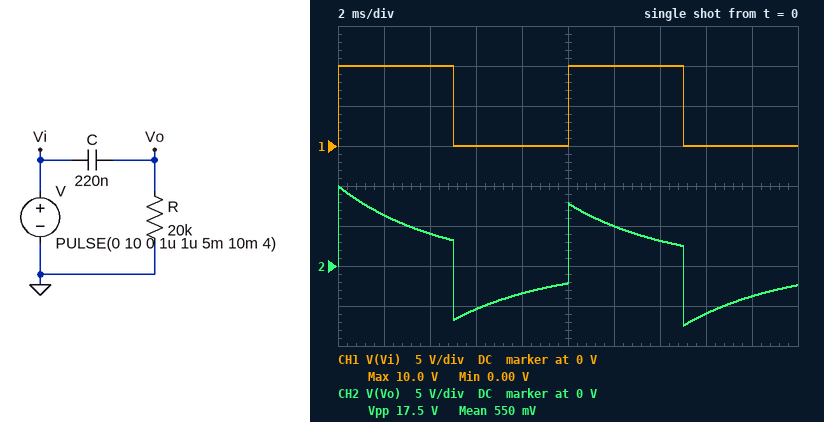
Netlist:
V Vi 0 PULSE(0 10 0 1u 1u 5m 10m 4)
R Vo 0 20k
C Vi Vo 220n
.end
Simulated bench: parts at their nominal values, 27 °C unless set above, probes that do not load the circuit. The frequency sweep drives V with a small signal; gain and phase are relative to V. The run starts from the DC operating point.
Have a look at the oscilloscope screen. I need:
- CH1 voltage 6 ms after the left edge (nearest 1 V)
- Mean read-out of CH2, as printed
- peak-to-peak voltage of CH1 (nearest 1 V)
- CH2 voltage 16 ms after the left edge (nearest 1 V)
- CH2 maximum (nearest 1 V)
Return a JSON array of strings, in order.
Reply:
["0 V", "550 mV", "10 V", "-6 V", "10 V"]
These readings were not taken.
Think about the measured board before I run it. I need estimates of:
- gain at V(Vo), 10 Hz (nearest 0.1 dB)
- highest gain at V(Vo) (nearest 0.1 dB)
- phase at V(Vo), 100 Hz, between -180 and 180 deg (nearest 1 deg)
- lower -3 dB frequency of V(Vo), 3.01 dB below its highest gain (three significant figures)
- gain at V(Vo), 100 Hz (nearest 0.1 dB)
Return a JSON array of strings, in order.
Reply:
["-11.5 dB", "0 dB", "20 deg", "36.2 Hz", "-0.5 dB"]
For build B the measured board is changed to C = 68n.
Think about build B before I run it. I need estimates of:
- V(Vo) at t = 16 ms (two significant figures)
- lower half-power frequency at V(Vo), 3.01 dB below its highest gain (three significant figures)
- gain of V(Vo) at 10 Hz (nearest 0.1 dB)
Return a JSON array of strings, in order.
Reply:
["-4.7 V", "117 Hz", "-21.4 dB"]
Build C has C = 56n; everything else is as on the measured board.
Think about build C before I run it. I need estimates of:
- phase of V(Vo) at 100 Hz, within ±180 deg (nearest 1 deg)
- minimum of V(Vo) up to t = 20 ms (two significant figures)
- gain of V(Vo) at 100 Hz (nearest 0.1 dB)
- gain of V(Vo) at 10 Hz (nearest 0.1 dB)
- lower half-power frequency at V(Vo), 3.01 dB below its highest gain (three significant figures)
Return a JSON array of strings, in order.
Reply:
["55 deg", "-9.9 V", "-4.8 dB", "-23.1 dB", "142 Hz"]
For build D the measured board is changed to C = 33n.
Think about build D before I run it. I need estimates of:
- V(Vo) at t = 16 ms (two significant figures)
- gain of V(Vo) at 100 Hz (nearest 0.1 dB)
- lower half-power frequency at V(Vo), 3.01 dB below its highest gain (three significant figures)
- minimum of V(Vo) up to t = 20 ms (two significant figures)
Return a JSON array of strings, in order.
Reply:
["-2.2 V", "-8.3 dB", "241 Hz", "-10 V"]
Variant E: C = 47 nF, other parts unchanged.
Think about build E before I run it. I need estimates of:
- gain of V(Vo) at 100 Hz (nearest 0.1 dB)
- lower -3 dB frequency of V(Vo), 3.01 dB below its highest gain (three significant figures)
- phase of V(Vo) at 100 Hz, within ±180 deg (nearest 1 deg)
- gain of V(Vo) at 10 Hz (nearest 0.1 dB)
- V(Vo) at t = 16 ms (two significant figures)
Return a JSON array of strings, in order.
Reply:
["-5.9 dB", "169 Hz", "59 deg", "-24.6 dB", "-3.4 V"]
